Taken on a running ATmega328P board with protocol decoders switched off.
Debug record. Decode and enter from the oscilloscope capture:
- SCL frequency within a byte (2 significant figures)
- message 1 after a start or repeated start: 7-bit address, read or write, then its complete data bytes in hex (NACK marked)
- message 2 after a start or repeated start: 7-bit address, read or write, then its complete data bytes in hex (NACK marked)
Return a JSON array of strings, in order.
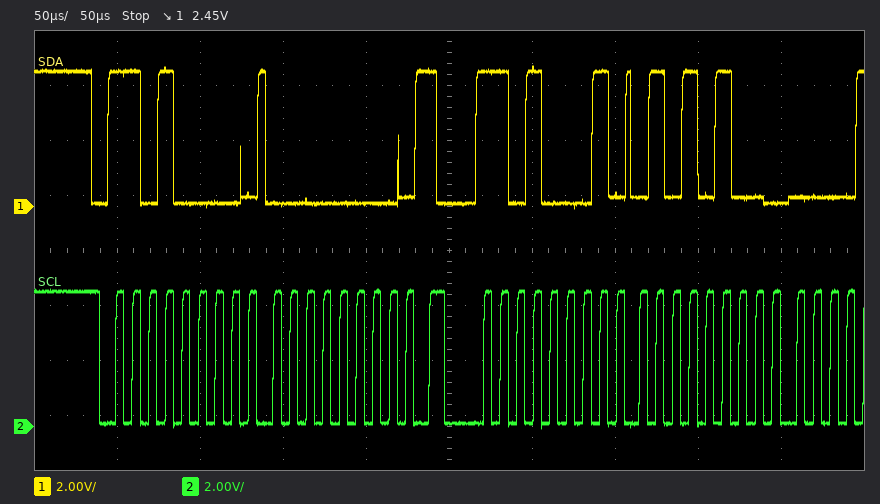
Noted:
["100 kHz", "0x68 write: 00", "0x68 read: 54"]
